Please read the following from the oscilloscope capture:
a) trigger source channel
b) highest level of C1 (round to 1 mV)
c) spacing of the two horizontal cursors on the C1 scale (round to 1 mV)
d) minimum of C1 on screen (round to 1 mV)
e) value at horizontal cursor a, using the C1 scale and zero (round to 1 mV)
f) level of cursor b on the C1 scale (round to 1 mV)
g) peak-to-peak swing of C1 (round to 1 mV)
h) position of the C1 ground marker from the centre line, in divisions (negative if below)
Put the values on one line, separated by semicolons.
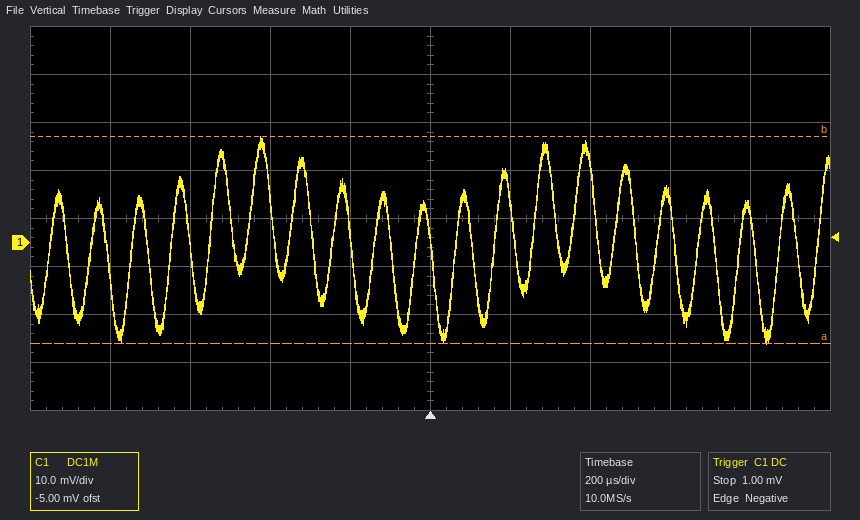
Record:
C1; 22 mV; 43 mV; -21 mV; -21 mV; 22 mV; 43 mV; -0.5 div
